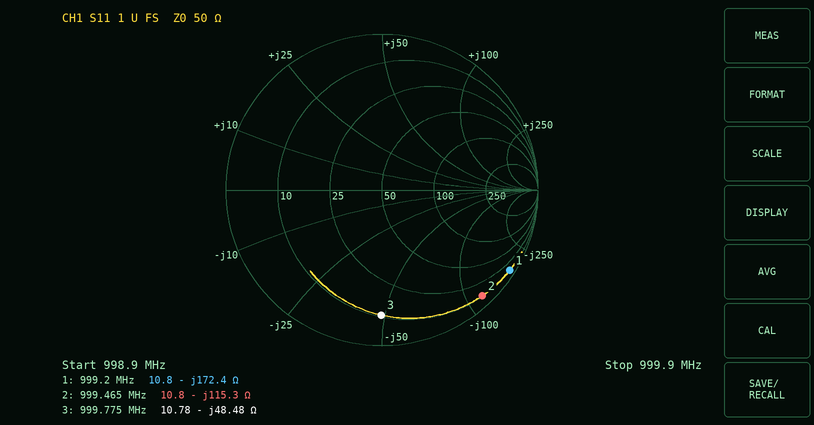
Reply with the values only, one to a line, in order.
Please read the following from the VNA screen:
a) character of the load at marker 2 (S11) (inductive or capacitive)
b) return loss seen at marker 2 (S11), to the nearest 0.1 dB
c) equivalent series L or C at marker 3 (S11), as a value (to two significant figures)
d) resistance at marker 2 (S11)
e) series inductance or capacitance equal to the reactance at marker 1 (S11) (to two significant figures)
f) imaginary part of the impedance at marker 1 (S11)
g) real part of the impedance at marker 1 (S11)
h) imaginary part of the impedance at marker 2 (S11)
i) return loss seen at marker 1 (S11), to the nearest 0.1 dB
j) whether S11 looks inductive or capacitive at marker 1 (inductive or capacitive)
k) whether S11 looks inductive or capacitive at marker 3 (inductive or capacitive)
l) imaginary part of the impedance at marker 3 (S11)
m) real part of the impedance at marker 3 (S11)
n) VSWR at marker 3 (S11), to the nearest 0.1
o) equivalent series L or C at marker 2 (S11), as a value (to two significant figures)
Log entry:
capacitive
0.6 dB
3.3 pF
10.8 Ω
920 fF
-172.4 Ω
10.8 Ω
-115.3 Ω
0.3 dB
capacitive
capacitive
-48.48 Ω
10.78 Ω
9.1
1.4 pF
